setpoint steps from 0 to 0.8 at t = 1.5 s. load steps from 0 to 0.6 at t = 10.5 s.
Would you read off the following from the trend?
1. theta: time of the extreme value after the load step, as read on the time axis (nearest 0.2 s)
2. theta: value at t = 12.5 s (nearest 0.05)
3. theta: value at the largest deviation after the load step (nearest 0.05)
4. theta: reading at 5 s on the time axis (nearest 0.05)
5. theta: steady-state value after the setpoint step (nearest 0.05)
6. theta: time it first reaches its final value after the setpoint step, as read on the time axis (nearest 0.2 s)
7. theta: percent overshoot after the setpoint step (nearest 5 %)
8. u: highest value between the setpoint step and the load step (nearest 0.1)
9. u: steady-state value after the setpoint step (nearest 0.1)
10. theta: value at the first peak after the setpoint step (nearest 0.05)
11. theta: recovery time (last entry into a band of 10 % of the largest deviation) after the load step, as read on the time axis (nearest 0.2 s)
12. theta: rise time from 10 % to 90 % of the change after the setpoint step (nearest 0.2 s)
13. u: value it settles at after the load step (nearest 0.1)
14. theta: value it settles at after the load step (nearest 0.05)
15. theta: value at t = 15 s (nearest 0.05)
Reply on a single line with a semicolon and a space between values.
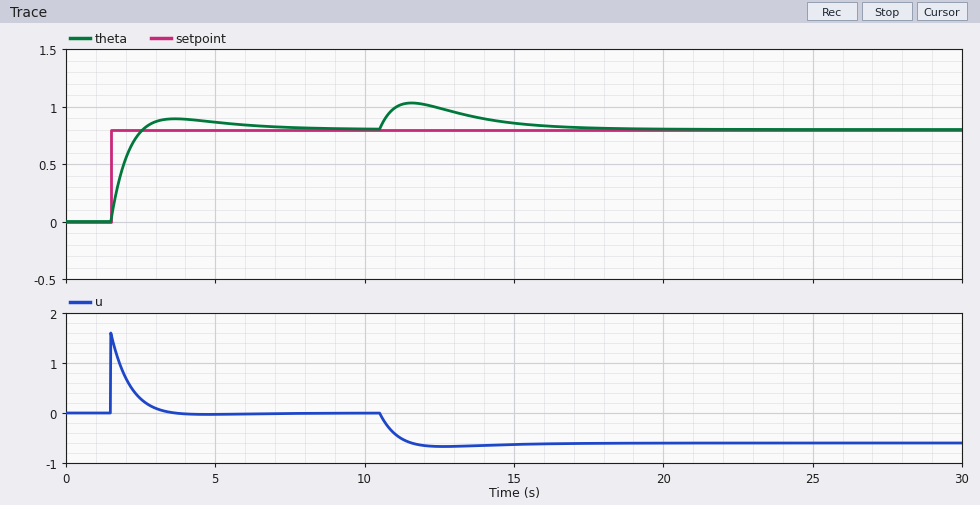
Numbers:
11.6 s; 1.00; 1.05; 0.85; 0.80; 2.6 s; 10 %; 1.6; 0.0; 0.90; 16.6 s; 0.8 s; -0.6; 0.80; 0.85
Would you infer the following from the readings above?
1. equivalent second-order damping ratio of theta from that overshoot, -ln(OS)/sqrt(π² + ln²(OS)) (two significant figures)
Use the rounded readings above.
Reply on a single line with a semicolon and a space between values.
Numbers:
0.59
